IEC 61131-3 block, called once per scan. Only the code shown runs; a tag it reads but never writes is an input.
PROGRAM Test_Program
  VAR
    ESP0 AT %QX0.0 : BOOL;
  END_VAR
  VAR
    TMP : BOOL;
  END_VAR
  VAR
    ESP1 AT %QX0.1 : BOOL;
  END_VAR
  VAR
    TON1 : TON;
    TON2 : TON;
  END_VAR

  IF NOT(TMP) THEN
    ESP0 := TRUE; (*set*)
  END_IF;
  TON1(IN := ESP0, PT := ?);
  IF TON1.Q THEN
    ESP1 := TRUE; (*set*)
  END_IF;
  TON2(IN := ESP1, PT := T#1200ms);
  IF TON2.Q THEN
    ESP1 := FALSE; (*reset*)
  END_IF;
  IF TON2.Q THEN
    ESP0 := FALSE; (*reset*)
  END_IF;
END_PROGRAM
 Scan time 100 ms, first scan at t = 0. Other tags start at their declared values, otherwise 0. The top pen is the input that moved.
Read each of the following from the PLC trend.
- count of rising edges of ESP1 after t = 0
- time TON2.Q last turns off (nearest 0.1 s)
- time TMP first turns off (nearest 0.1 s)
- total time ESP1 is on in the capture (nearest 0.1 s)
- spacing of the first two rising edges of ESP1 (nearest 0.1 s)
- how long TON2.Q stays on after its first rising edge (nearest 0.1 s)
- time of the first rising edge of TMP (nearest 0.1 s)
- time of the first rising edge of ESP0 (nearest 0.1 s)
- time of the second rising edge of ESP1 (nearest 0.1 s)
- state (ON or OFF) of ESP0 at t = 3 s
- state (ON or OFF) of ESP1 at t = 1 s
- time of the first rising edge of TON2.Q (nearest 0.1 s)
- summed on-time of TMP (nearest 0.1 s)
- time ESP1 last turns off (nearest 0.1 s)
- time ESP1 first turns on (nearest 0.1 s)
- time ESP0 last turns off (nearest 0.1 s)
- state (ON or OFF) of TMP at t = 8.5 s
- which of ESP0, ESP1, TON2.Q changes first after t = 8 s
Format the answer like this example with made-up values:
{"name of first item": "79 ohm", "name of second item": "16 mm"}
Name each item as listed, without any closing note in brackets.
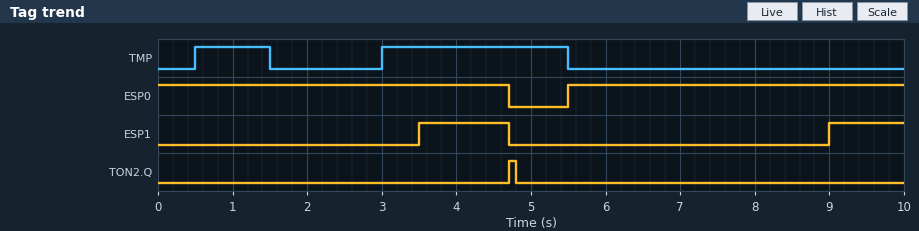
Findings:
{"count of rising edges of ESP1 after t = 0": "2", "time TON2.Q last turns off": "4.8 s", "time TMP first turns off": "1.5 s", "total time ESP1 is on in the capture": "2.2 s", "spacing of the first two rising edges of ESP1": "5.5 s", "how long TON2.Q stays on after its first rising edge": "0.1 s", "time of the first rising edge of TMP": "0.5 s", "time of the first rising edge of ESP0": "5.5 s", "time of the second rising edge of ESP1": "9.0 s", "state (ON or OFF) of ESP0 at t = 3 s": "ON", "state (ON or OFF) of ESP1 at t = 1 s": "OFF", "time of the first rising edge of TON2.Q": "4.7 s", "summed on-time of TMP": "3.5 s", "time ESP1 last turns off": "4.7 s", "time ESP1 first turns on": "3.5 s", "time ESP0 last turns off": "4.7 s", "state (ON or OFF) of TMP at t = 8.5 s": "OFF", "which of ESP0, ESP1, TON2.Q changes first after t = 8 s": "ESP1"}
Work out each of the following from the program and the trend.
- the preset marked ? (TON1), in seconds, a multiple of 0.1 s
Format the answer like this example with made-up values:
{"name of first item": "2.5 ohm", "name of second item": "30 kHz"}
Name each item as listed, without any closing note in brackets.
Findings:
{"the preset marked ? (TON1), in seconds, a multiple of 0.1 s": "3.5 s"}
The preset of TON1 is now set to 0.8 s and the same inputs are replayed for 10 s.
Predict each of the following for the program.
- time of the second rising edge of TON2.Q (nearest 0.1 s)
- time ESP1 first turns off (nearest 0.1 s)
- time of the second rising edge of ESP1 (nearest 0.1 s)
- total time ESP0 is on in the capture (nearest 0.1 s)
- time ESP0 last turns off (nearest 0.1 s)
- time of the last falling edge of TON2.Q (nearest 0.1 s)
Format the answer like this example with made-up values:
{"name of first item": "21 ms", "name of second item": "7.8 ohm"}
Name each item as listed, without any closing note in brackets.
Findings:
{"time of the second rising edge of TON2.Q": "7.5 s", "time ESP1 first turns off": "2.0 s", "time of the second rising edge of ESP1": "6.3 s", "total time ESP0 is on in the capture": "4.0 s", "time ESP0 last turns off": "7.5 s", "time of the last falling edge of TON2.Q": "3.0 s"}
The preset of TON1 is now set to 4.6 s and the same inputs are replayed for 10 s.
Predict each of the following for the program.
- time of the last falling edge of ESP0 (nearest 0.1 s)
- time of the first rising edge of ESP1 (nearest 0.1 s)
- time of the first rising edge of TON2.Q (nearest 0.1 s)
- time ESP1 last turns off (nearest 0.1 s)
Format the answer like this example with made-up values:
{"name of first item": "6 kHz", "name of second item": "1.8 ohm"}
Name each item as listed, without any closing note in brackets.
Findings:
{"time of the last falling edge of ESP0": "5.8 s", "time of the first rising edge of ESP1": "4.6 s", "time of the first rising edge of TON2.Q": "5.8 s", "time ESP1 last turns off": "5.8 s"}
